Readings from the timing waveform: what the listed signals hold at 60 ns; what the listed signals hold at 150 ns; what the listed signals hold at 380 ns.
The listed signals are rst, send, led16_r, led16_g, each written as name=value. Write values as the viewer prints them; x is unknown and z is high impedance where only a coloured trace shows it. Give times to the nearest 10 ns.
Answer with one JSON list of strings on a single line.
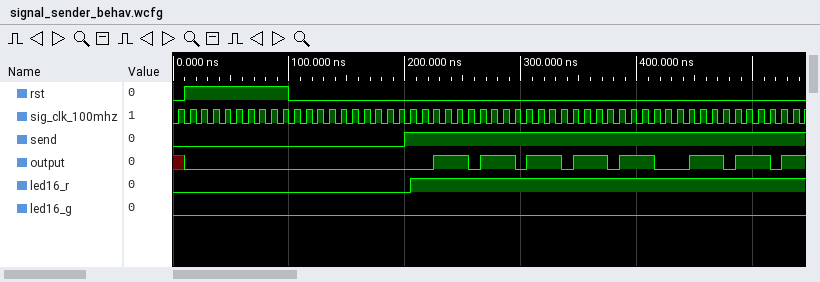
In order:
["rst=1, send=0, led16_r=0, led16_g=0", "rst=0, send=0, led16_r=0, led16_g=0", "rst=0, send=1, led16_r=1, led16_g=0"]
